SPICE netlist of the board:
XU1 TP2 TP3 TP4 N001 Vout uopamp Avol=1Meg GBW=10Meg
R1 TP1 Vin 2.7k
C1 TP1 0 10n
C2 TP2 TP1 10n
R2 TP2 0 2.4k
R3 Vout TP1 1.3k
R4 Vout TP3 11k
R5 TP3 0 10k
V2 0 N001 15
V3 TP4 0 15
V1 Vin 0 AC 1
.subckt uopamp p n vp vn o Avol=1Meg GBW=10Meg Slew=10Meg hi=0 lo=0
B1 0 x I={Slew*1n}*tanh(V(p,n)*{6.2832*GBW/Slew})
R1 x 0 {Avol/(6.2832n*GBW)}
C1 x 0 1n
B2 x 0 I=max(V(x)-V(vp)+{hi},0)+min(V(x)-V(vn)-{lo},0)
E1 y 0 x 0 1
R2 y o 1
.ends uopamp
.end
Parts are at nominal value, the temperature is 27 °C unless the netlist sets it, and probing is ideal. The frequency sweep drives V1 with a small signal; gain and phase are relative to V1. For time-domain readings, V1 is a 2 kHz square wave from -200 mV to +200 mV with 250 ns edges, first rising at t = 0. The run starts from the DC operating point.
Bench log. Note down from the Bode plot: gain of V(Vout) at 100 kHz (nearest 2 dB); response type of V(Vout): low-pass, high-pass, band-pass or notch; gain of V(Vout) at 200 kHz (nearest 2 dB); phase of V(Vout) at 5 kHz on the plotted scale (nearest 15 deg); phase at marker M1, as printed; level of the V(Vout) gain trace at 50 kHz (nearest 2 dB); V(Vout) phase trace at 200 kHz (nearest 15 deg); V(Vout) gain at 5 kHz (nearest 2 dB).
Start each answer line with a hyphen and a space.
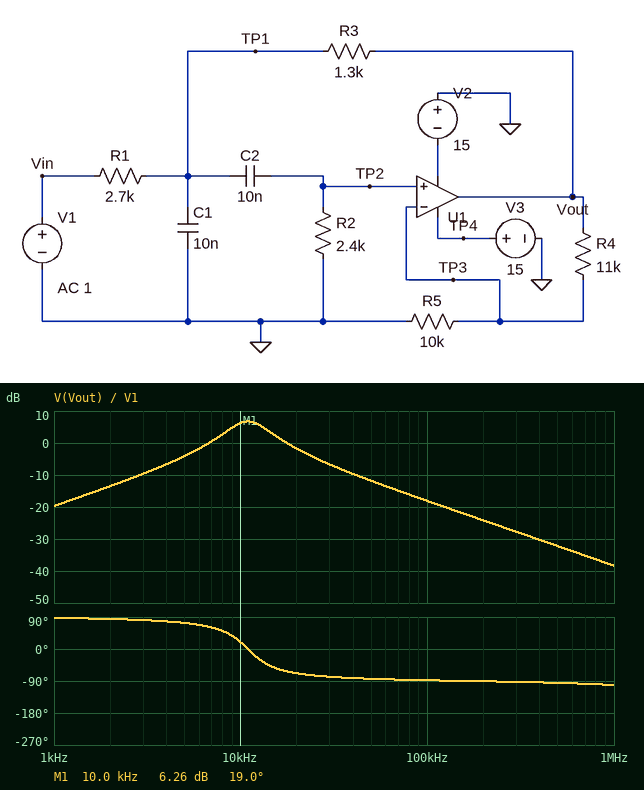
- -18 dB
- band-pass
- -24 dB
- 75 deg
- 19.0 deg
- -12 dB
- -90 deg
- -4 dB
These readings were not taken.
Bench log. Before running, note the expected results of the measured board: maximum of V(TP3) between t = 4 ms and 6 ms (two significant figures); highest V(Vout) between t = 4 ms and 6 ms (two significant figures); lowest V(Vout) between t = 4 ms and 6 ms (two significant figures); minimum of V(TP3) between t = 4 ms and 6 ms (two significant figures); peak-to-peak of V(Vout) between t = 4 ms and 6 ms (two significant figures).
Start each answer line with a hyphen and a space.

- 150 mV
- 320 mV
- -320 mV
- -150 mV
- 640 mV
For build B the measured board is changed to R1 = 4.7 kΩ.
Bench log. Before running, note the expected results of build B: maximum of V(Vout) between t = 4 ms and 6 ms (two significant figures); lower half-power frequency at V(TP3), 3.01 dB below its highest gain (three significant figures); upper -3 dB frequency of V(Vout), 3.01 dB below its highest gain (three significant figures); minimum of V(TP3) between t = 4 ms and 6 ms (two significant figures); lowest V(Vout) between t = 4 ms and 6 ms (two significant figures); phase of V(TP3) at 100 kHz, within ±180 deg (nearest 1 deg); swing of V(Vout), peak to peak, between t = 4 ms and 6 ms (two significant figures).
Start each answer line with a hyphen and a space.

- 240 mV
- 8.69 kHz
- 11.9 kHz
- -120 mV
- -240 mV
- -89 deg
- 490 mV
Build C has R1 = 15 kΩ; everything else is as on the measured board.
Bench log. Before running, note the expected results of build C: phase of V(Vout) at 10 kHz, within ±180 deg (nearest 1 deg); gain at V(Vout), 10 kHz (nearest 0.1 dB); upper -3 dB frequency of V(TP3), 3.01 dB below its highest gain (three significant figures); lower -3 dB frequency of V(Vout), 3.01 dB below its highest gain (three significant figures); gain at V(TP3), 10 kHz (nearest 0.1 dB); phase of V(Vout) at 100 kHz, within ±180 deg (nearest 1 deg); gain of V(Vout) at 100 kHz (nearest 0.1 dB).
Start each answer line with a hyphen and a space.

- -55 deg
- 3.4 dB
- 9.80 kHz
- 8.95 kHz
- -3.0 dB
- -91 deg
- -33.0 dB
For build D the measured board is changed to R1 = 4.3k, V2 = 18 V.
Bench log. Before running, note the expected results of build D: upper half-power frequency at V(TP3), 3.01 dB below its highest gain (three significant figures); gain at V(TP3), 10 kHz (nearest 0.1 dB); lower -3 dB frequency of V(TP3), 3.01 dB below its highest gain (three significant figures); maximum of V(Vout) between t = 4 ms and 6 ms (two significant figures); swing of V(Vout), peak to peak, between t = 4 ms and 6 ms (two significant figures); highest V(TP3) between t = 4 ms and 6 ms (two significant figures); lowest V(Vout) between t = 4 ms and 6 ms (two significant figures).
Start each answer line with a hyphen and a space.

- 12.1 kHz
- 0.4 dB
- 8.66 kHz
- 250 mV
- 510 mV
- 120 mV
- -250 mV
